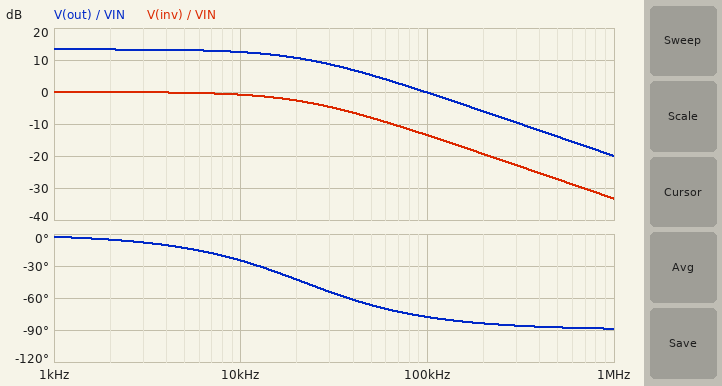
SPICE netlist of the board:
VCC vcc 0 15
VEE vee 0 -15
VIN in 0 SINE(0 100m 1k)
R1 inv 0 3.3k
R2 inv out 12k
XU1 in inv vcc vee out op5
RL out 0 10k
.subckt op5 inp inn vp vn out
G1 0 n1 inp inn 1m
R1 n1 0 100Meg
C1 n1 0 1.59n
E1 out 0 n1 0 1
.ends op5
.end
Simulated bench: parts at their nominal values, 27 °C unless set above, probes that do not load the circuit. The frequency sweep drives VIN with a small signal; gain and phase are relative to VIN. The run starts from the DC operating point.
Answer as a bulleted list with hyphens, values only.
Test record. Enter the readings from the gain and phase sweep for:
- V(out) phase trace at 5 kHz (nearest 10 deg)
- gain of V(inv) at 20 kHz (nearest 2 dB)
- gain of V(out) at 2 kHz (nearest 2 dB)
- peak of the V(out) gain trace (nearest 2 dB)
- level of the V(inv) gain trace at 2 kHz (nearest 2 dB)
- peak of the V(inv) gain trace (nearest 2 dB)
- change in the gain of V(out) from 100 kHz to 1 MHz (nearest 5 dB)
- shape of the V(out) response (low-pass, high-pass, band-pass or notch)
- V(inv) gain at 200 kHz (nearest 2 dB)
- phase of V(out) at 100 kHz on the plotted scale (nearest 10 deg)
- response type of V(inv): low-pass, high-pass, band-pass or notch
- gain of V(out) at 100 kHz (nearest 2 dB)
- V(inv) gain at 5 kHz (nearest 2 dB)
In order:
- -10 deg
- -2 dB
- 14 dB
- 14 dB
- 0 dB
- 0 dB
- -20 dB
- low-pass
- -20 dB
- -80 deg
- low-pass
- 0 dB
- 0 dB
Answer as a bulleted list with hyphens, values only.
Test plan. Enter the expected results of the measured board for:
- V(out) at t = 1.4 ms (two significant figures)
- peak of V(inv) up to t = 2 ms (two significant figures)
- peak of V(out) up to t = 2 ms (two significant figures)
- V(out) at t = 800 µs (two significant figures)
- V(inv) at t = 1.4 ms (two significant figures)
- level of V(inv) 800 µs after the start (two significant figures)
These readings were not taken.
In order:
- 290 mV
- 100 mV
- 460 mV
- -450 mV
- 62 mV
- -96 mV
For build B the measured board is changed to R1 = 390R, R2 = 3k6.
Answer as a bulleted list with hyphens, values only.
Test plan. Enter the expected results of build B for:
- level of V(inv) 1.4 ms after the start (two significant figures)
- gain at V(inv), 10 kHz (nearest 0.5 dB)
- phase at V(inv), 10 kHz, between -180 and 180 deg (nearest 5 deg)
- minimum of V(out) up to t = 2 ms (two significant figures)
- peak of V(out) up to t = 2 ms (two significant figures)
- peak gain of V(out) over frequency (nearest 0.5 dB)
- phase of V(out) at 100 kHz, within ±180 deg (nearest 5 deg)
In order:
- 66 mV
- -3.0 dB
- -45 deg
- -1.0 V
- 1.0 V
- 20.0 dB
- -85 deg
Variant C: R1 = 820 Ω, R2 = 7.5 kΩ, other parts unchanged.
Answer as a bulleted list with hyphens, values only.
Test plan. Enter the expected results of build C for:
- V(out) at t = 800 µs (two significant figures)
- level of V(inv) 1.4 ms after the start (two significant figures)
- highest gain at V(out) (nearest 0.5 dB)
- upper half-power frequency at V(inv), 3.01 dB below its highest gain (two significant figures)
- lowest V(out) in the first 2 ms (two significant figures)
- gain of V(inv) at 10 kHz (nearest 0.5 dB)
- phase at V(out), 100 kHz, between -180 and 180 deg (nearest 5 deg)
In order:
- -990 mV
- 66 mV
- 20.0 dB
- 9.9 kHz
- -1.0 V
- -3.0 dB
- -85 deg
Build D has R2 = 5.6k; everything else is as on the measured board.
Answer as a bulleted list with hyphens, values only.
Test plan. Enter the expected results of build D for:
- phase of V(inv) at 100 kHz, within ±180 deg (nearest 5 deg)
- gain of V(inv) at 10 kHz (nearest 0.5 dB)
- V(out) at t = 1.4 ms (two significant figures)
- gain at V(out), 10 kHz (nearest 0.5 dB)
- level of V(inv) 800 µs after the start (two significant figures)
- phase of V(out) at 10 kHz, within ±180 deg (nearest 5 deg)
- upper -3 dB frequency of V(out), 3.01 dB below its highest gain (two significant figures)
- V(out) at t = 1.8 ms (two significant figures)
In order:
- -70 deg
- -0.5 dB
- 160 mV
- 8.5 dB
- -96 mV
- -15 deg
- 37 kHz
- -260 mV
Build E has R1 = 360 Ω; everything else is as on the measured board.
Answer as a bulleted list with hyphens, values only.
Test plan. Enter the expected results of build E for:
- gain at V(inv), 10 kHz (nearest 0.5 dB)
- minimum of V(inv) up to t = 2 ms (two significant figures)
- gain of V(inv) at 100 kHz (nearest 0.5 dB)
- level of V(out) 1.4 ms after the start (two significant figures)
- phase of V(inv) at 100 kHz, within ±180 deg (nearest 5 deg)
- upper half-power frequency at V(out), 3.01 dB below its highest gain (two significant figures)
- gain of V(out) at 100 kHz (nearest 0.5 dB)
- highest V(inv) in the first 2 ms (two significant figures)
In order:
- -11.0 dB
- -95 mV
- -30.5 dB
- 2.7 V
- -90 deg
- 2.9 kHz
- 0 dB
- 95 mV
